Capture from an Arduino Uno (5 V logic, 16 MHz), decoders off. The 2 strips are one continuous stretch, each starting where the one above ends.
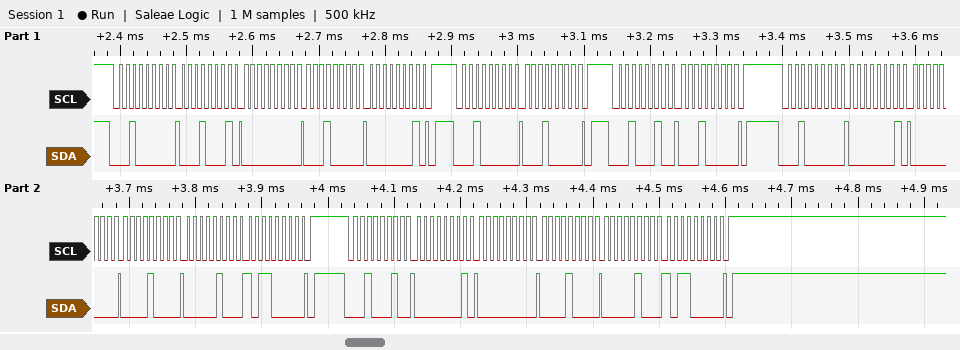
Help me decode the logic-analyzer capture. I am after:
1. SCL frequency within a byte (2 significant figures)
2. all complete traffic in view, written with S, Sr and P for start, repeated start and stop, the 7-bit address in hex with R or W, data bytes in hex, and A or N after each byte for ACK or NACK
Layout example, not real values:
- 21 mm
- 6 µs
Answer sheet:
- 100 kHz
- S 10W A 11 A 00 A 10 A 01 A P S 10W A 10 A P S 11W A 10 A P S 10W A 01 A 00 A 08 A 04 A B0 A P S 11W A 01 A 00 A 08 A 04 A B0 A P
